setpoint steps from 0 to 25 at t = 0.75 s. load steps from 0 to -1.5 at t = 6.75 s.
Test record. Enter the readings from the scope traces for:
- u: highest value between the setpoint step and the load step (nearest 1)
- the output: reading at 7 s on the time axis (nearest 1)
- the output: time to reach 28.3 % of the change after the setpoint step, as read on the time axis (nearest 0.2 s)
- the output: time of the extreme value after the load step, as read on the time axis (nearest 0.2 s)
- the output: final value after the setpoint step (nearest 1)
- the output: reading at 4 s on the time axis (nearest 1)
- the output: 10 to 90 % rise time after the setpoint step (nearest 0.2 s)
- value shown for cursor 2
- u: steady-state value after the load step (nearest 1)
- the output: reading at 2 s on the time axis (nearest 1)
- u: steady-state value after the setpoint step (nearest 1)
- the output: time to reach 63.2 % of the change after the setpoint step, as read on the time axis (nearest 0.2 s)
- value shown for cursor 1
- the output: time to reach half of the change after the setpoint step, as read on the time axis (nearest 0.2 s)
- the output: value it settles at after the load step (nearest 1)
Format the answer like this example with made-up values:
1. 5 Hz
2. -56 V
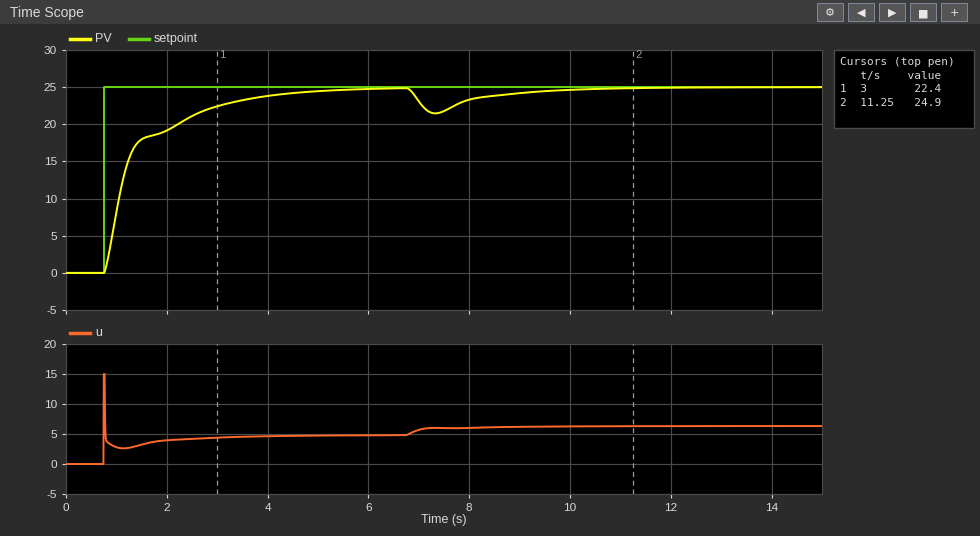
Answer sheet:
1. 15
2. 23
3. 1.0 s
4. 7.4 s
5. 25
6. 24
7. 2.2 s
8. 24.9
9. 6
10. 19
11. 5
12. 1.2 s
13. 22.4
14. 1.2 s
15. 25
